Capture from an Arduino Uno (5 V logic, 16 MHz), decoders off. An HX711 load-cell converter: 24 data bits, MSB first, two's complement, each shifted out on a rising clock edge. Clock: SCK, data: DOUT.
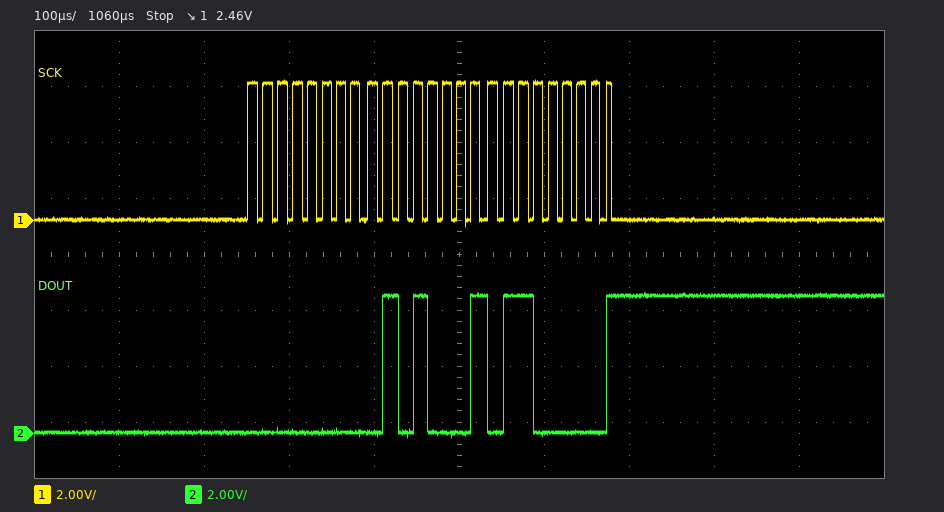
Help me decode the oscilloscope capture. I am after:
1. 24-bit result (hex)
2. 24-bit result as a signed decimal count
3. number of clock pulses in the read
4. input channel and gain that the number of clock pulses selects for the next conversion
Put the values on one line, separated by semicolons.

0x005160; 20832; 25; channel A, gain 128
